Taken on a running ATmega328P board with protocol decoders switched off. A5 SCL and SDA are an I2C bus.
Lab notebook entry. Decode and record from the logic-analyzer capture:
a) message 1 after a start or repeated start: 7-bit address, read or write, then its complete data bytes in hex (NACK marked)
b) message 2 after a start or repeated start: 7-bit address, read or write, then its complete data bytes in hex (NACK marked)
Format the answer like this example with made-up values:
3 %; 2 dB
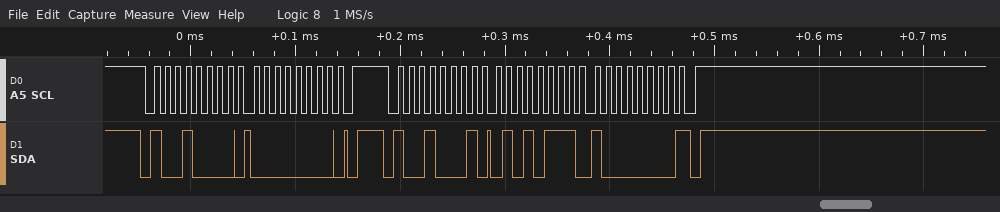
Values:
0x48 write: 00; 0x48 read: 57 80 NACK
